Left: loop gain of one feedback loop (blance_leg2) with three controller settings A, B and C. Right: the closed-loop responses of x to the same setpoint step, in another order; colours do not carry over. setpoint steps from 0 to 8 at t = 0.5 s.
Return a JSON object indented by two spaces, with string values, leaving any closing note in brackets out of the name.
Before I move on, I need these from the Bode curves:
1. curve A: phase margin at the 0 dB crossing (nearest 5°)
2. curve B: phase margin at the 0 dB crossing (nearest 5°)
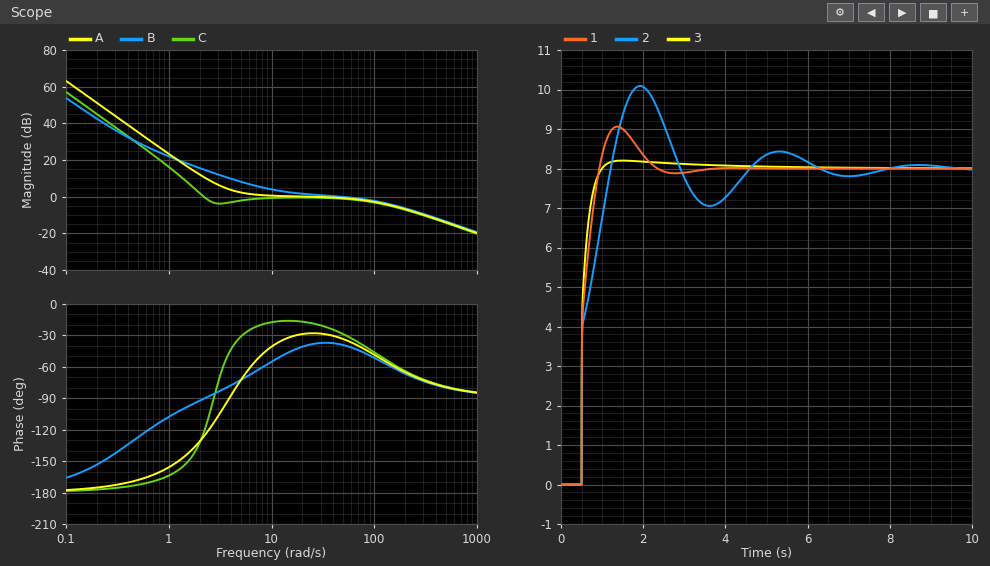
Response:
{
  "curve A: phase margin at the 0 dB crossing": "150°",
  "curve B: phase margin at the 0 dB crossing": "140°"
}
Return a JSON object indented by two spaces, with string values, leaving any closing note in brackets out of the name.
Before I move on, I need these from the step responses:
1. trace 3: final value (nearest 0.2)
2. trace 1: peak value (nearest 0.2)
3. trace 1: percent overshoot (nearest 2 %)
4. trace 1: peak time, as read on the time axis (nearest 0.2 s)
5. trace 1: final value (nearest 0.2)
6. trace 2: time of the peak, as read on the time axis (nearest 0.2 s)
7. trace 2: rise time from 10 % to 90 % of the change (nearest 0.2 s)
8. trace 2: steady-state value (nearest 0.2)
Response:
{
  "trace 3: final value": "8.0",
  "trace 1: peak value": "9.0",
  "trace 1: percent overshoot": "14 %",
  "trace 1: peak time, as read on the time axis": "1.4 s",
  "trace 1: final value": "8.0",
  "trace 2: time of the peak, as read on the time axis": "2.0 s",
  "trace 2: rise time from 10 % to 90 % of the change": "0.6 s",
  "trace 2: steady-state value": "8.0"
}
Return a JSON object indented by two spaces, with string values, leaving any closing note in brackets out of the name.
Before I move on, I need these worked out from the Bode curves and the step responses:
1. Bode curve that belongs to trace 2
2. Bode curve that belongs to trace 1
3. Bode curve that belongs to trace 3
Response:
{
  "Bode curve that belongs to trace 2": "C",
  "Bode curve that belongs to trace 1": "A",
  "Bode curve that belongs to trace 3": "B"
}
